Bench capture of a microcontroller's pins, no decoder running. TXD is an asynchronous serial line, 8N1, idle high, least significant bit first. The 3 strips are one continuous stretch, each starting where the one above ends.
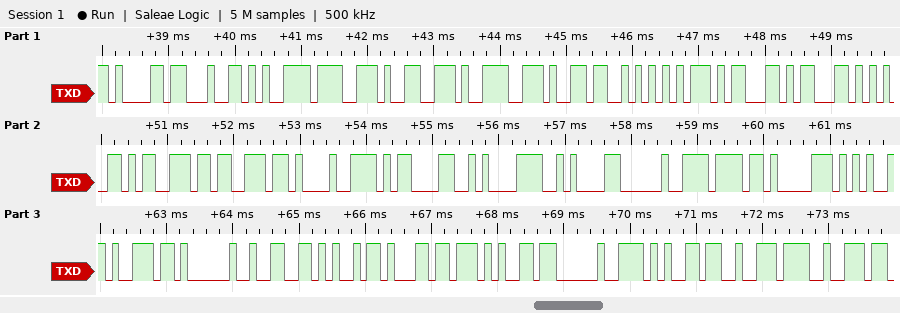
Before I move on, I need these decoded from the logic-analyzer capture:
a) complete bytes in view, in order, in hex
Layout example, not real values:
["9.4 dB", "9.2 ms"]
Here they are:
["61 64 79 2E 2E 2E 53 75 63 63 65 73 73 21 0D 0A 0A 20 6F 70 65 6E 20 66 69 6C 65 20 65 72 72"]
